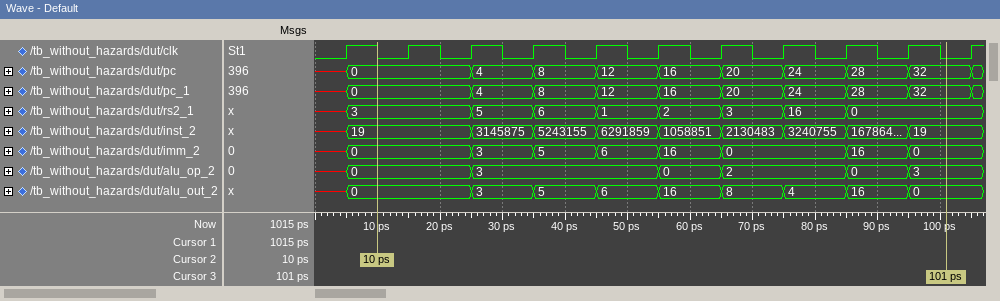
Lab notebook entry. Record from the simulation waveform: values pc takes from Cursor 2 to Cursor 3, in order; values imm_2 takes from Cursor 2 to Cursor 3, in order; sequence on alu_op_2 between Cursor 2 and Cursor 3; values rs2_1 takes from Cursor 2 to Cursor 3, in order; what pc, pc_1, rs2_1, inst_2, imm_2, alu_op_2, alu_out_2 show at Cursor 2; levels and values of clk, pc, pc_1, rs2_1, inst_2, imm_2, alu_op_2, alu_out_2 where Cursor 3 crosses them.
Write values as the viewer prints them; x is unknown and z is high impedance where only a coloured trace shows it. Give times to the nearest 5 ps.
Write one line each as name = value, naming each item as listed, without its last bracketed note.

values pc takes from Cursor 2 to Cursor 3, in order = 0, 4, 8, 12, 16, 20, 24, 28, 32
values imm_2 takes from Cursor 2 to Cursor 3, in order = 0, 3, 5, 6, 16, 0, 16, 0
sequence on alu_op_2 between Cursor 2 and Cursor 3 = 0, 3, 0, 2, 0, 3
values rs2_1 takes from Cursor 2 to Cursor 3, in order = 3, 5, 6, 1, 2, 3, 16, 0
what pc, pc_1, rs2_1, inst_2, imm_2, alu_op_2, alu_out_2 show at Cursor 2 = pc=0, pc_1=0, rs2_1=3, inst_2=19, imm_2=0, alu_op_2=0, alu_out_2=0
levels and values of clk, pc, pc_1, rs2_1, inst_2, imm_2, alu_op_2, alu_out_2 where Cursor 3 crosses them = clk=0, pc=32, pc_1=32, rs2_1=0, inst_2=19, imm_2=0, alu_op_2=3, alu_out_2=0
